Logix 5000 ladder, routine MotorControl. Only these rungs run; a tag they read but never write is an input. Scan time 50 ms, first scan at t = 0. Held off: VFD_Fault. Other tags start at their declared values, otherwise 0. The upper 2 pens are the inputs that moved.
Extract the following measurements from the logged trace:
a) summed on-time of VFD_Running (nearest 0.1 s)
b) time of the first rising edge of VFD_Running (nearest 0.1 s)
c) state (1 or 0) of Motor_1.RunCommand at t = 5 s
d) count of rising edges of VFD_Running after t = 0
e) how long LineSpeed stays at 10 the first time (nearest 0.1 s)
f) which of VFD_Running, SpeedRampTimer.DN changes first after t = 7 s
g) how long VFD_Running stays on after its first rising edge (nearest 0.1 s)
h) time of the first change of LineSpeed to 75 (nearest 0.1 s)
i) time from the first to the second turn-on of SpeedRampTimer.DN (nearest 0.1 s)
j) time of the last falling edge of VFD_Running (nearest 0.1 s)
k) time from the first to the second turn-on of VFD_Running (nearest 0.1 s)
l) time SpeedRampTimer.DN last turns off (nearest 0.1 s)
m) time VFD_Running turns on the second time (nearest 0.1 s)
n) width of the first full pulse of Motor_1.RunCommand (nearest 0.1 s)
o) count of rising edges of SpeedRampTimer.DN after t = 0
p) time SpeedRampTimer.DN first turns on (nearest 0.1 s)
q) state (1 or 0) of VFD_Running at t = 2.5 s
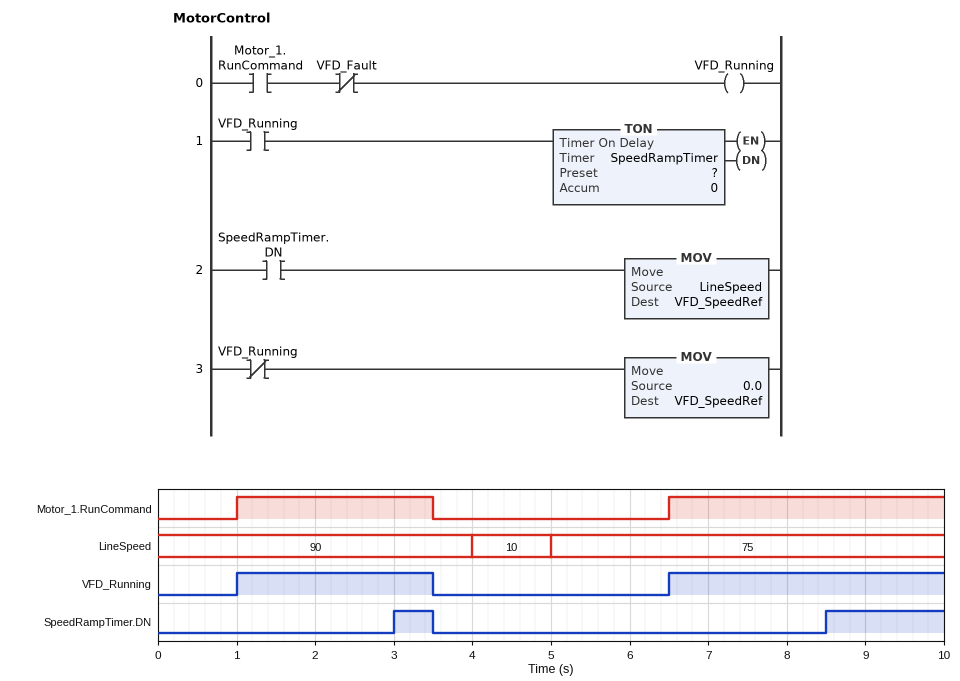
6.0 s
1.0 s
0
2
1.0 s
SpeedRampTimer.DN
2.5 s
5.0 s
5.5 s
3.5 s
5.5 s
3.5 s
6.5 s
2.5 s
2
3.0 s
1
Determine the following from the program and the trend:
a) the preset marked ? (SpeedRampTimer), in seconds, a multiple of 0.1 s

2.0 s
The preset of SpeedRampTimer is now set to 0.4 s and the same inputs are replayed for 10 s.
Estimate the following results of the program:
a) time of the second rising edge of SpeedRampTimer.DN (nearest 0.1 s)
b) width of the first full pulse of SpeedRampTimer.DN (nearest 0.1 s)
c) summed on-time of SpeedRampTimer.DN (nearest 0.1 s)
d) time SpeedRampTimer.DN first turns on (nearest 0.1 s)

6.9 s
2.1 s
5.2 s
1.4 s
